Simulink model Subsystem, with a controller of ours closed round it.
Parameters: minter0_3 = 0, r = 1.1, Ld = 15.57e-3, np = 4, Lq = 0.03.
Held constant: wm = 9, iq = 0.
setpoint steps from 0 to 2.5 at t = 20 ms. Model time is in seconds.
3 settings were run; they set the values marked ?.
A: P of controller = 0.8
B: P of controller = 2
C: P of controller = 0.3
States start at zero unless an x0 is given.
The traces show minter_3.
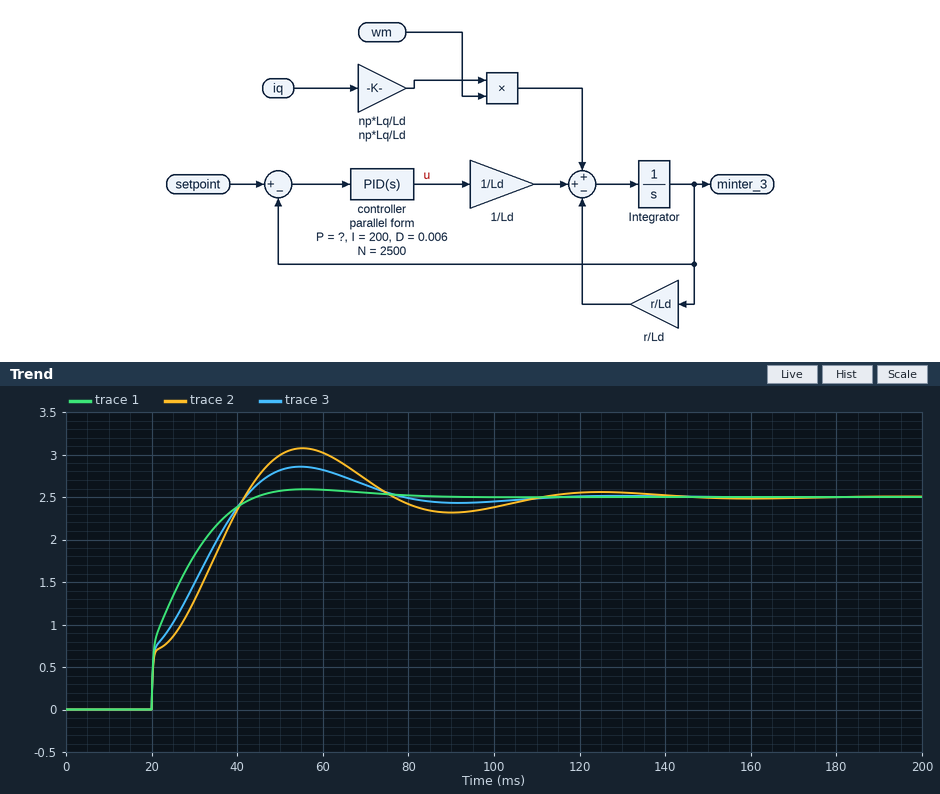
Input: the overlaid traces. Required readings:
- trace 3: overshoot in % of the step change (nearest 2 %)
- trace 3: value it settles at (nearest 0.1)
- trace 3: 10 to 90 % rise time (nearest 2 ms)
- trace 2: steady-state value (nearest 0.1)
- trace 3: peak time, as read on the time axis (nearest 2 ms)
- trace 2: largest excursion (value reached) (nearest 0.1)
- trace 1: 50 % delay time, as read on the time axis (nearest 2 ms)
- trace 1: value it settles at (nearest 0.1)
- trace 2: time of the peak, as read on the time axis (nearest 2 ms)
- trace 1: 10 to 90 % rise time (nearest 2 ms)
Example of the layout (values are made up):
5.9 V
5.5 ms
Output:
14 %
2.5
18 ms
2.5
54 ms
3.1
24 ms
2.5
56 ms
16 ms
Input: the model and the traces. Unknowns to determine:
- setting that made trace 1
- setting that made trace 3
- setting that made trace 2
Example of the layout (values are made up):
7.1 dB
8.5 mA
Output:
B
A
C
